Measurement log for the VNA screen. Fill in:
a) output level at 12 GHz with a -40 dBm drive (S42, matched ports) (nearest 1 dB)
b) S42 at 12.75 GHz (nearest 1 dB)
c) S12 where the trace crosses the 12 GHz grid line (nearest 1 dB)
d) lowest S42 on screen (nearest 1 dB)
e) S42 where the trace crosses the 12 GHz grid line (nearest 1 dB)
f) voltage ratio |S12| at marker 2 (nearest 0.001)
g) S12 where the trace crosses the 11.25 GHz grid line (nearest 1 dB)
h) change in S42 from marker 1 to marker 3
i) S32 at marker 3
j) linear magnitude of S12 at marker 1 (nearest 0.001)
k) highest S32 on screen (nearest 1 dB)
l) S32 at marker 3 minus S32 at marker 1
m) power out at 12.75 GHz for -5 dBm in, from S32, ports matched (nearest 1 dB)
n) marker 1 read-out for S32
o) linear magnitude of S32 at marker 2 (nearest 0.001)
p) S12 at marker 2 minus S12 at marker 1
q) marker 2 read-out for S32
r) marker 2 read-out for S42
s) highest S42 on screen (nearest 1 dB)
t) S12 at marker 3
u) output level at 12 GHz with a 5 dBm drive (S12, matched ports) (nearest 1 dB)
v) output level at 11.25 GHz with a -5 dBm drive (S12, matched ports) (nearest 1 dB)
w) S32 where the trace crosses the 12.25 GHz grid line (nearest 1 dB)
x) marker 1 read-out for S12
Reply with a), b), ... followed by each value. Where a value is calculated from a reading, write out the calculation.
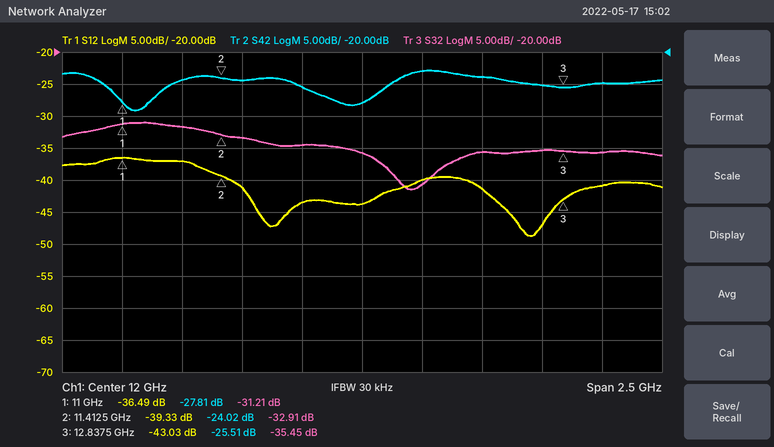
a) -40 dBm + (-28 dB) = -68 dBm
b) -25 dB
c) -44 dB
d) -29 dB
e) -28 dB
f) 10^(-39.33/20) ≈ 0.011
g) -37 dB
h) -25.51 − (-27.81) = 2.30 dB
i) -35.45 dB
j) 10^(-36.49/20) ≈ 0.015
k) -31 dB
l) -35.45 − (-31.21) = -4.24 dB
m) -5 dBm + (-35 dB) = -40 dBm
n) -31.21 dB
o) 10^(-32.91/20) ≈ 0.023
p) -39.33 − (-36.49) = -2.84 dB
q) -32.91 dB
r) -24.02 dB
s) -23 dB
t) -43.03 dB
u) 5 dBm + (-44 dB) = -39 dBm
v) -5 dBm + (-37 dB) = -42 dBm
w) -41 dB
x) -36.49 dB
